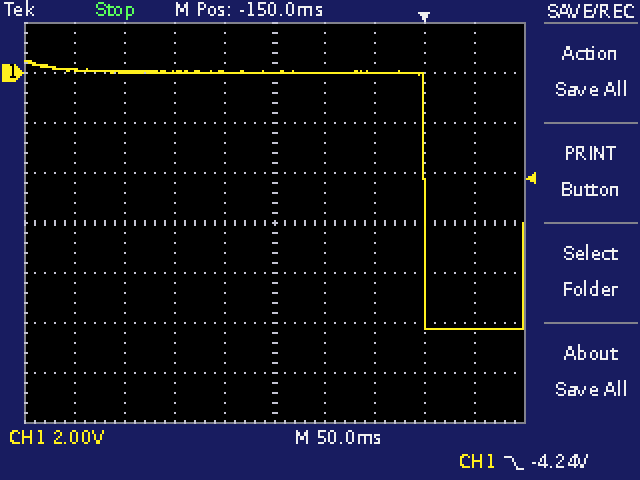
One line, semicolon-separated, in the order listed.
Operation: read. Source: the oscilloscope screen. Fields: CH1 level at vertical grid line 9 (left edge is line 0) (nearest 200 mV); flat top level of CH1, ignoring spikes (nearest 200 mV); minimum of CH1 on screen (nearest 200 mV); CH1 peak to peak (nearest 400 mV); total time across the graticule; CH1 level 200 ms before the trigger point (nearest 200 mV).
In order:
-10.2 V; 0.0 V; -10.2 V; 10.8 V; 500 ms; 0.0 V
